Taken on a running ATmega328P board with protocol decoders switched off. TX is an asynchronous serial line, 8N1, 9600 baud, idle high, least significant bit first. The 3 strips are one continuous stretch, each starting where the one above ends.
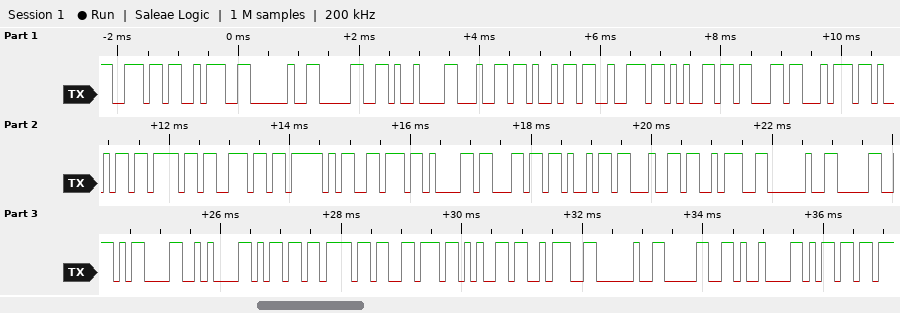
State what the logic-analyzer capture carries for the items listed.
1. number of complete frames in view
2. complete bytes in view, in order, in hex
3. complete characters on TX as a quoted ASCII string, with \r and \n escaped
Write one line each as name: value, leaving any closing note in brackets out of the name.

number of complete frames in view: 34
complete bytes in view, in order, in hex: 0x6E 0x3A 0x20 0x30 0x09 0x64 0x69 0x72 0x65 0x63 0x74 0x69 0x6F 0x6E 0x5F 0x76 0x61 0x6C 0x69 0x64 0x3A 0x20 0x30 0x0D 0x0A 0x6D 0x6F 0x76 0x65 0x3A 0x20 0x30 0x09 0x6D
complete characters on TX as a quoted ASCII string, with \r and \n escaped: "n: 0\tdirection_valid: 0\r\nmove: 0\tm"
